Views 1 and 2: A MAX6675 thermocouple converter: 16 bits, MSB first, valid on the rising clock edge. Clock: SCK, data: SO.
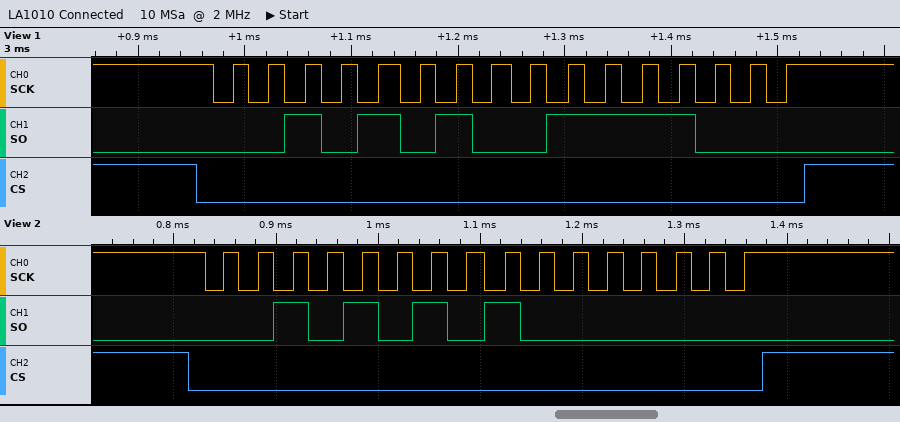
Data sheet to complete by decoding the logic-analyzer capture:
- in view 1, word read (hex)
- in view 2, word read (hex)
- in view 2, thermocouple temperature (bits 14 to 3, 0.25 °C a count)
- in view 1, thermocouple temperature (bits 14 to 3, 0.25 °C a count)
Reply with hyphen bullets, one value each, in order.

- 0x2A78
- 0x2A80
- 340.00 °C
- 339.75 °C
